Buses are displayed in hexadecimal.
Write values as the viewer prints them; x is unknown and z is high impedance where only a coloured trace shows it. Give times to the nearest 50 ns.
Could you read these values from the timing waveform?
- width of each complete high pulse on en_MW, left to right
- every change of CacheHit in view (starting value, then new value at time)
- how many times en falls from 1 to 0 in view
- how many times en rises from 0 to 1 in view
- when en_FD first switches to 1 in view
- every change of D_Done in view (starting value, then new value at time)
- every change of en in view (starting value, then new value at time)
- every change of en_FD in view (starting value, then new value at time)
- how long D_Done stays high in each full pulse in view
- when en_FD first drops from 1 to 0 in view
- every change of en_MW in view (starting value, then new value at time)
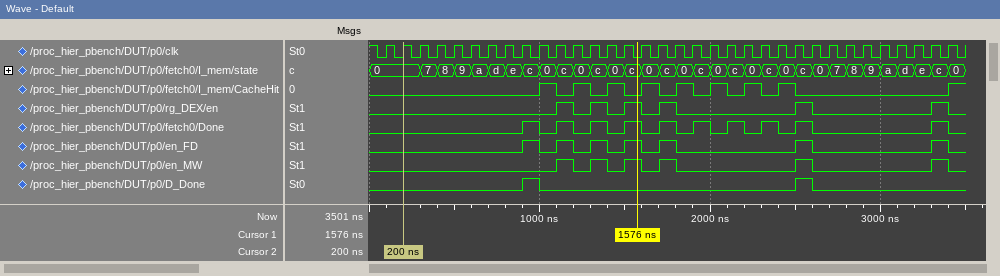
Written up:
100 ns, 100 ns, 100 ns, 100 ns, 100 ns, 100 ns
0, 1 at 1000 ns, 0 at 1100 ns, 1 at 1200 ns, 0 at 1300 ns, 1 at 1400 ns, 0 at 1500 ns, 1 at 1600 ns, 0 at 1700 ns, 1 at 1800 ns, 0 at 1900 ns, 1 at 2000 ns, 0 at 2100 ns, 1 at 2200 ns, 0 at 2300 ns, 1 at 2400 ns, 0 at 2500 ns, 1 at 3400 ns
6
6
900 ns
0, 1 at 900 ns, 0 at 1000 ns, 1 at 2500 ns, 0 at 2600 ns
0, 1 at 1100 ns, 0 at 1200 ns, 1 at 1300 ns, 0 at 1400 ns, 1 at 1500 ns, 0 at 1600 ns, 1 at 1700 ns, 0 at 1800 ns, 1 at 2500 ns, 0 at 2600 ns, 1 at 3300 ns, 0 at 3400 ns
0, 1 at 900 ns, 0 at 1000 ns, 1 at 1100 ns, 0 at 1200 ns, 1 at 1300 ns, 0 at 1400 ns, 1 at 1500 ns, 0 at 1600 ns, 1 at 1700 ns, 0 at 1800 ns, 1 at 2500 ns, 0 at 2600 ns, 1 at 3300 ns, 0 at 3400 ns
100 ns, 100 ns
1000 ns
0, 1 at 1100 ns, 0 at 1200 ns, 1 at 1300 ns, 0 at 1400 ns, 1 at 1500 ns, 0 at 1600 ns, 1 at 1700 ns, 0 at 1800 ns, 1 at 2500 ns, 0 at 2600 ns, 1 at 3300 ns, 0 at 3400 ns
